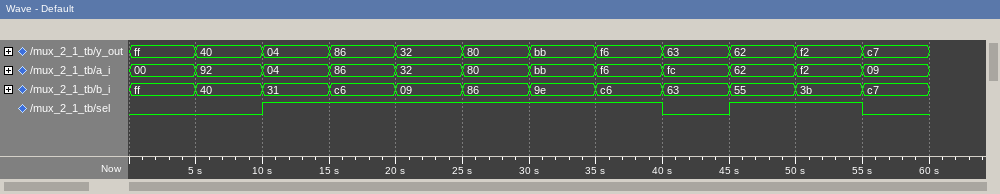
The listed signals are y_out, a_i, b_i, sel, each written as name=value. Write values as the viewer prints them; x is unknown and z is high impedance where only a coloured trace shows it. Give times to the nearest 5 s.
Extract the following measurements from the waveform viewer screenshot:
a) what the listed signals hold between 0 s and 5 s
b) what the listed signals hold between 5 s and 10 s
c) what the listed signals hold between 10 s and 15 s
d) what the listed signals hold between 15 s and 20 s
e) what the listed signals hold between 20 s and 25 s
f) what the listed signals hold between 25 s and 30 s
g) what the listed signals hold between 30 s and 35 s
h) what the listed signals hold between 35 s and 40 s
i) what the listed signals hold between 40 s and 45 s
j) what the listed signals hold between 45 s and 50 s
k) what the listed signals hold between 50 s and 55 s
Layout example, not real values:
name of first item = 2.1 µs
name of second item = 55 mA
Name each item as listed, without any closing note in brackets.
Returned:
what the listed signals hold between 0 s and 5 s = y_out=ff, a_i=00, b_i=ff, sel=0
what the listed signals hold between 5 s and 10 s = y_out=40, a_i=92, b_i=40, sel=0
what the listed signals hold between 10 s and 15 s = y_out=04, a_i=04, b_i=31, sel=1
what the listed signals hold between 15 s and 20 s = y_out=86, a_i=86, b_i=c6, sel=1
what the listed signals hold between 20 s and 25 s = y_out=32, a_i=32, b_i=09, sel=1
what the listed signals hold between 25 s and 30 s = y_out=80, a_i=80, b_i=86, sel=1
what the listed signals hold between 30 s and 35 s = y_out=bb, a_i=bb, b_i=9e, sel=1
what the listed signals hold between 35 s and 40 s = y_out=f6, a_i=f6, b_i=c6, sel=1
what the listed signals hold between 40 s and 45 s = y_out=63, a_i=fc, b_i=63, sel=0
what the listed signals hold between 45 s and 50 s = y_out=62, a_i=62, b_i=55, sel=1
what the listed signals hold between 50 s and 55 s = y_out=f2, a_i=f2, b_i=3b, sel=1
